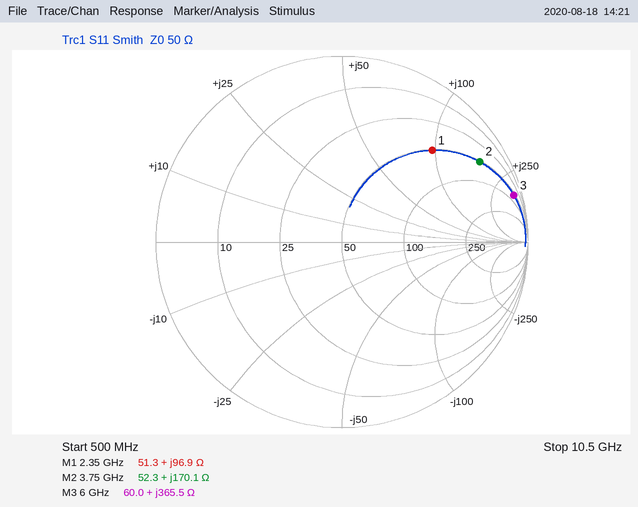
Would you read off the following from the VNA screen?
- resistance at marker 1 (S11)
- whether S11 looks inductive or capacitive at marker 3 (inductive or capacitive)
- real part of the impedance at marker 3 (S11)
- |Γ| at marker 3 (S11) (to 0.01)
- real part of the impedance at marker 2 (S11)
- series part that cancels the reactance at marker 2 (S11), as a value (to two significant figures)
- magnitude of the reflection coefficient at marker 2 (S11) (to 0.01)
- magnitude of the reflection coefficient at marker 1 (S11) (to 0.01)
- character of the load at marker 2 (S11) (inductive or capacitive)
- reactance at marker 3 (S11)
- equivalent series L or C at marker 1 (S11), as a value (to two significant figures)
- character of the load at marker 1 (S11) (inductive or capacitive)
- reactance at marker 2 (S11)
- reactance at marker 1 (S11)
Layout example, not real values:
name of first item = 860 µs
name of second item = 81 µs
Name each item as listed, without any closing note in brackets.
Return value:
resistance at marker 1 = 51.3 Ω
whether S11 looks inductive or capacitive at marker 3 = inductive
real part of the impedance at marker 3 = 60.0 Ω
|Γ| at marker 3 (S11) = 0.96
real part of the impedance at marker 2 = 52.3 Ω
series part that cancels the reactance at marker 2 (S11), as a value = 250 fF
magnitude of the reflection coefficient at marker 2 (S11) = 0.86
magnitude of the reflection coefficient at marker 1 (S11) = 0.69
character of the load at marker 2 (S11) = inductive
reactance at marker 3 = +365.5 Ω
equivalent series L or C at marker 1 (S11), as a value = 6.6 nH
character of the load at marker 1 (S11) = inductive
reactance at marker 2 = +170.1 Ω
reactance at marker 1 = +96.9 Ω
